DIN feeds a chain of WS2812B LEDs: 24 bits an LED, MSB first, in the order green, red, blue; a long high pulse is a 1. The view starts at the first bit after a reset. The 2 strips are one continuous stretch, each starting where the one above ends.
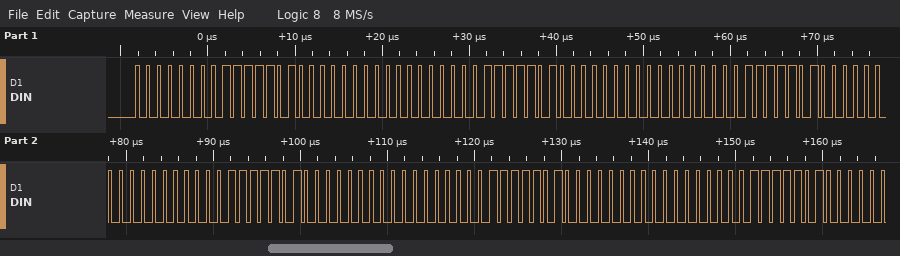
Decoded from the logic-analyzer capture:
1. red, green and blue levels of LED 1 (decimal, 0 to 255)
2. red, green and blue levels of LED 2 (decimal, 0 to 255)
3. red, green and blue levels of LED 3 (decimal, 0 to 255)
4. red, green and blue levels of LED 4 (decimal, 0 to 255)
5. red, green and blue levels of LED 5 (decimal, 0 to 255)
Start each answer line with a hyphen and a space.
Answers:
- 250, 0, 0
- 250, 0, 0
- 250, 0, 0
- 250, 0, 0
- 250, 0, 0
